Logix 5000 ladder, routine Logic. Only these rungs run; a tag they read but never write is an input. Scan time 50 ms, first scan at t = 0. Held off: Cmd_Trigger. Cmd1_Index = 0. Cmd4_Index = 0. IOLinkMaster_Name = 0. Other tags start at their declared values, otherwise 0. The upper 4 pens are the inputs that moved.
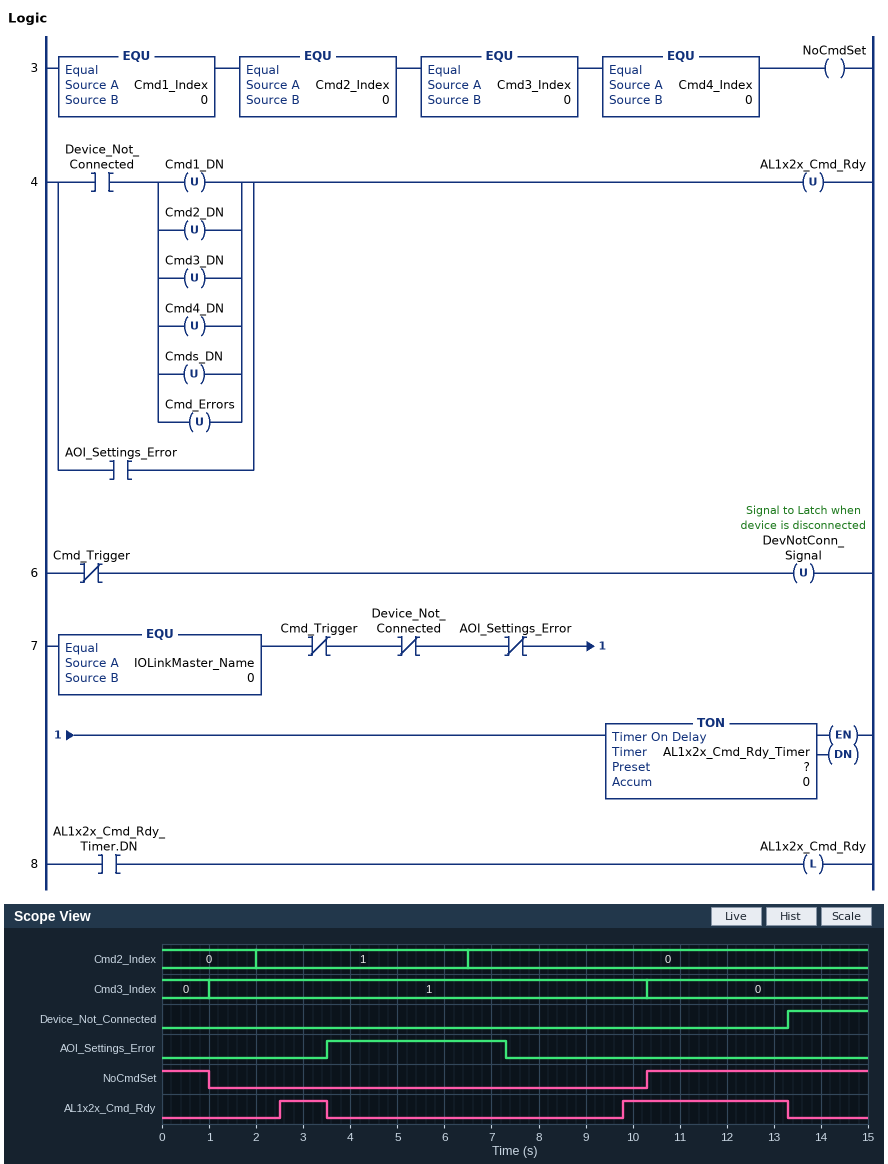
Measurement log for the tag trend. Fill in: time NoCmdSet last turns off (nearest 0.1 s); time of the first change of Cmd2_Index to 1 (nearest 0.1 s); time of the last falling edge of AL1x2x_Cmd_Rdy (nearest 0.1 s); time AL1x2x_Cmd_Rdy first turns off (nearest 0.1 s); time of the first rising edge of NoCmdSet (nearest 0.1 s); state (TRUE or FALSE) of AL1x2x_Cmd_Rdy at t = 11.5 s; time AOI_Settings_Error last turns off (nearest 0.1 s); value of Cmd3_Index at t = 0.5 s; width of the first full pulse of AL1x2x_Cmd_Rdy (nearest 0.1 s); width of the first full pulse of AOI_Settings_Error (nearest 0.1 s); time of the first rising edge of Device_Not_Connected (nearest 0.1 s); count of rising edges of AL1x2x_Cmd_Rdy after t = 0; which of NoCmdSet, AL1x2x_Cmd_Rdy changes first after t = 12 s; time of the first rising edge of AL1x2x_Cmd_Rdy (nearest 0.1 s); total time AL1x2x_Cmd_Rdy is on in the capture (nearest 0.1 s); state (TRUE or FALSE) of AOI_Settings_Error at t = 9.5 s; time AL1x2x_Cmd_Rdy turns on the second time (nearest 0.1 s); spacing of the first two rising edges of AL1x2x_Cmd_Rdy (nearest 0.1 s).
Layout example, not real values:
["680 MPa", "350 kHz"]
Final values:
["1.0 s", "2.0 s", "13.3 s", "3.5 s", "10.3 s", "TRUE", "7.3 s", "0", "1.0 s", "3.8 s", "13.3 s", "2", "AL1x2x_Cmd_Rdy", "2.5 s", "4.5 s", "FALSE", "9.8 s", "7.3 s"]
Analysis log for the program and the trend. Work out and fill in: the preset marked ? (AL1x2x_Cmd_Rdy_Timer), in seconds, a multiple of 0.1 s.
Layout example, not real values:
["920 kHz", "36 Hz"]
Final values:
["2.5 s"]
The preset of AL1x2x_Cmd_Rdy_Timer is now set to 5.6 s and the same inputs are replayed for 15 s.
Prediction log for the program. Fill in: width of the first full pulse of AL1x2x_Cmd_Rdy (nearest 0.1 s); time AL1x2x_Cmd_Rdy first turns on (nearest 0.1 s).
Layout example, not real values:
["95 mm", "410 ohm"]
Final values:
["0.4 s", "12.9 s"]
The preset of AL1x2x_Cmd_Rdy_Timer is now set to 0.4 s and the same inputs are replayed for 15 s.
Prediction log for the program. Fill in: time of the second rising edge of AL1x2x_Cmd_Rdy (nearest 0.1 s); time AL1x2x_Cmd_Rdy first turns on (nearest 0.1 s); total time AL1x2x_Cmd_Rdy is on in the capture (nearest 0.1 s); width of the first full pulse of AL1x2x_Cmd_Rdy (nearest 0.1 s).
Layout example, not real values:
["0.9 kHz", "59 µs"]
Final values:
["7.7 s", "0.4 s", "8.7 s", "3.1 s"]
